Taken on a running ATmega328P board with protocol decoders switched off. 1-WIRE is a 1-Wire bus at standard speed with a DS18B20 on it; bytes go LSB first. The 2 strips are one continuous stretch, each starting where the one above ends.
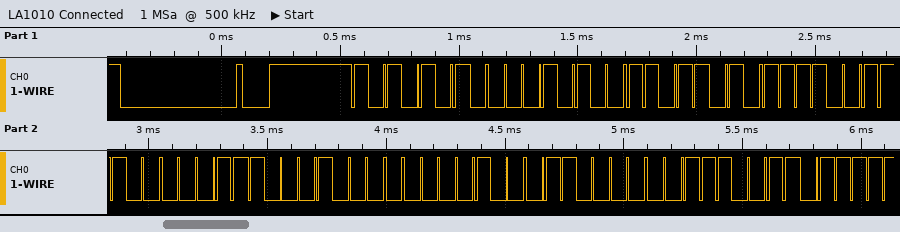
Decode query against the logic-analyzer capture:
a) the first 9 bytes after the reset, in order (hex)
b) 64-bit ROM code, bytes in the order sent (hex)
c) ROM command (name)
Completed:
55 28 5B CF C1 11 20 06 CE
28 5B CF C1 11 20 06 CE
Match ROM
